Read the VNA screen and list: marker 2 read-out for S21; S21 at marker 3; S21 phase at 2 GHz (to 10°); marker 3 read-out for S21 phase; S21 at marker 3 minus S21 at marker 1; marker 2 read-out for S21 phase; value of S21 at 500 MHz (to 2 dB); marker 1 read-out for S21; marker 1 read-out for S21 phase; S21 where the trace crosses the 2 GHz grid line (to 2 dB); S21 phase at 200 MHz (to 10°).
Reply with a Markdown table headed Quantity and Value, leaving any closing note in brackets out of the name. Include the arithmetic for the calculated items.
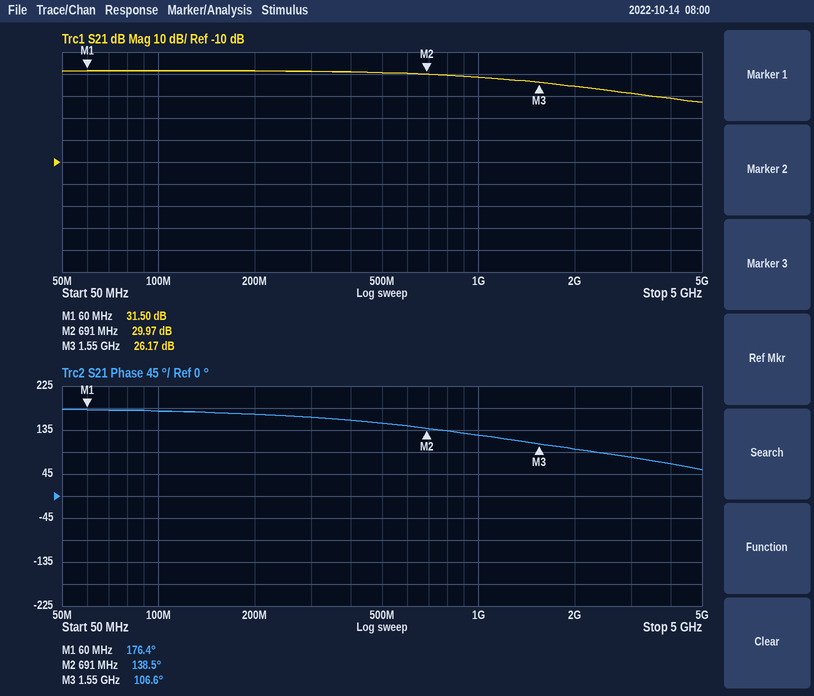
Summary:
| Quantity | Value |
|---|---|
| marker 2 read-out for S21 | 29.97 dB |
| S21 at marker 3 | 26.17 dB |
| S21 phase at 2 GHz | 100° |
| marker 3 read-out for S21 phase | 106.6° |
| S21 at marker 3 minus S21 at marker 1 | 26.17 − (31.5) = -5.33 dB |
| marker 2 read-out for S21 phase | 138.5° |
| value of S21 at 500 MHz | 30 dB |
| marker 1 read-out for S21 | 31.50 dB |
| marker 1 read-out for S21 phase | 176.4° |
| S21 where the trace crosses the 2 GHz grid line | 24 dB |
| S21 phase at 200 MHz | 170° |
